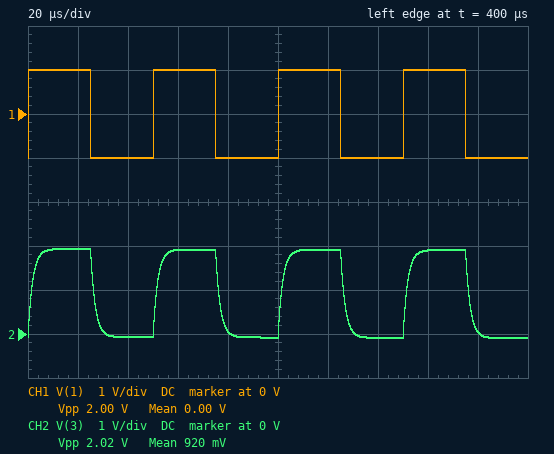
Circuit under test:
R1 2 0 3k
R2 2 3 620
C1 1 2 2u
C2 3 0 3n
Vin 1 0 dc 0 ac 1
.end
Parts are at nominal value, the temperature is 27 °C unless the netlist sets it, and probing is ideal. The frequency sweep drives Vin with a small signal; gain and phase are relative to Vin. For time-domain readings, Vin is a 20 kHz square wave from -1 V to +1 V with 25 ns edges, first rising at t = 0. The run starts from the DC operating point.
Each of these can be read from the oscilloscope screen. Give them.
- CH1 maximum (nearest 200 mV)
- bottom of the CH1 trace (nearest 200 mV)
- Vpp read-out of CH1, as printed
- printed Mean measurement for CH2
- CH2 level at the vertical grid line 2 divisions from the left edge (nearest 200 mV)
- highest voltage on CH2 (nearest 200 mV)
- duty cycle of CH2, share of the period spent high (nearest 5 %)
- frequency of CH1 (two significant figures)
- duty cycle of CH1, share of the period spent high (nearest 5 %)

1.0 V
-1.0 V
2.00 V
920 mV
0 V
2.0 V
50 %
20 kHz
50 %
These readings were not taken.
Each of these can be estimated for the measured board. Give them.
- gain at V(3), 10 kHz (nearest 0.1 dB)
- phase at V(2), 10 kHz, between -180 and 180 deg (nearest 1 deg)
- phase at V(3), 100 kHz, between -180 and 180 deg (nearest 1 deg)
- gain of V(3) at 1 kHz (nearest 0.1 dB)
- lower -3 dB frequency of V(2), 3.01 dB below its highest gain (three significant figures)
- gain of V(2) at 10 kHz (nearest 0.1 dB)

-0.1 dB
0 deg
-49 deg
0 dB
26.6 Hz
0 dB
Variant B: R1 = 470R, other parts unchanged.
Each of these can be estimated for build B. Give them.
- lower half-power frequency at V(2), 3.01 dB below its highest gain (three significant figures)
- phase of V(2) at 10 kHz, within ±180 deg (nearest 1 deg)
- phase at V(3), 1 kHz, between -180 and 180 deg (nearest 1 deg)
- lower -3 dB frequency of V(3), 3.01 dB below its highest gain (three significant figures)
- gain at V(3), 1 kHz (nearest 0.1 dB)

170 Hz
1 deg
9 deg
168 Hz
-0.1 dB
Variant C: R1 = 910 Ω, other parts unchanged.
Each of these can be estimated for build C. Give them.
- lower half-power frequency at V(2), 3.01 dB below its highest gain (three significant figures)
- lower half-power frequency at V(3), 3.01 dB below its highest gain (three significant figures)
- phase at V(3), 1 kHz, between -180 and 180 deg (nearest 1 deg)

87.6 Hz
87.1 Hz
4 deg
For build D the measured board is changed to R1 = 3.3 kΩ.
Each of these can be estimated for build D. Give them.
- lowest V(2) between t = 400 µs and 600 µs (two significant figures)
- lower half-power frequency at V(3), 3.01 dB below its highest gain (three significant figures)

-90 mV
24.1 Hz
